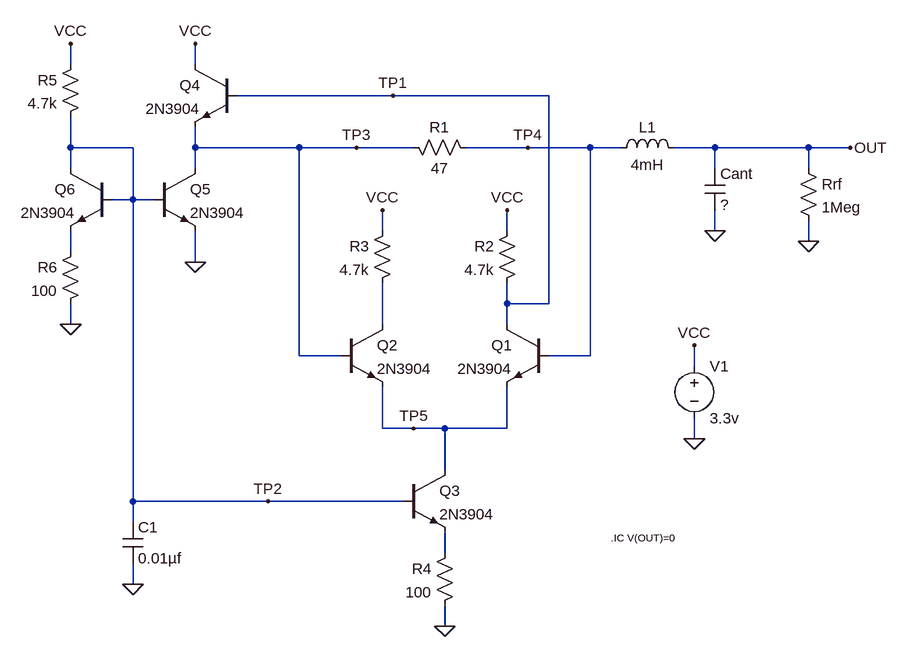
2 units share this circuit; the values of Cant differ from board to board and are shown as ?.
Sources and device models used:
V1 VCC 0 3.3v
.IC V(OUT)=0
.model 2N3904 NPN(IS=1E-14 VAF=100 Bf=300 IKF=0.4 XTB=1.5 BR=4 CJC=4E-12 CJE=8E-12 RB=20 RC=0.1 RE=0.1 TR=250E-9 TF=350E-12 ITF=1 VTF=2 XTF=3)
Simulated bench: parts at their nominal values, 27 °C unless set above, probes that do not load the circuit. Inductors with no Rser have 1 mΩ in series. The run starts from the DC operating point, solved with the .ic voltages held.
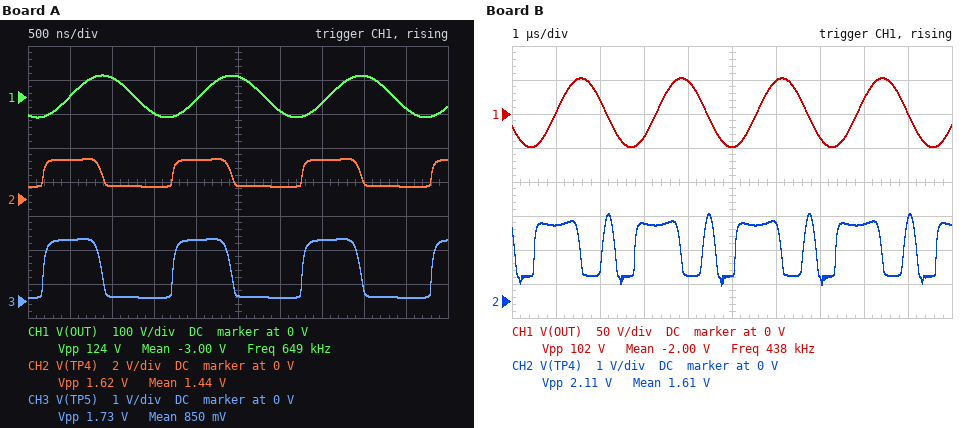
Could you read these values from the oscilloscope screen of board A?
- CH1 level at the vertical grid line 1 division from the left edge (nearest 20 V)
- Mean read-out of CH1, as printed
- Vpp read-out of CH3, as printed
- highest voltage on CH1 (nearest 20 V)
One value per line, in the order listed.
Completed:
0 V
-3.00 V
1.73 V
60 V
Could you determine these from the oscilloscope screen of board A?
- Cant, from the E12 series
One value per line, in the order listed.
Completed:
15 pF
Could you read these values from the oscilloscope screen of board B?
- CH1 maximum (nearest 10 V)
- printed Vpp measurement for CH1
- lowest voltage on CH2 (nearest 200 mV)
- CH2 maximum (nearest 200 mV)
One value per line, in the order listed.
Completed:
50 V
102 V
400 mV
2.6 V
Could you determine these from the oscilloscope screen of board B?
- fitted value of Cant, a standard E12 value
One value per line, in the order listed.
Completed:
33 pF
